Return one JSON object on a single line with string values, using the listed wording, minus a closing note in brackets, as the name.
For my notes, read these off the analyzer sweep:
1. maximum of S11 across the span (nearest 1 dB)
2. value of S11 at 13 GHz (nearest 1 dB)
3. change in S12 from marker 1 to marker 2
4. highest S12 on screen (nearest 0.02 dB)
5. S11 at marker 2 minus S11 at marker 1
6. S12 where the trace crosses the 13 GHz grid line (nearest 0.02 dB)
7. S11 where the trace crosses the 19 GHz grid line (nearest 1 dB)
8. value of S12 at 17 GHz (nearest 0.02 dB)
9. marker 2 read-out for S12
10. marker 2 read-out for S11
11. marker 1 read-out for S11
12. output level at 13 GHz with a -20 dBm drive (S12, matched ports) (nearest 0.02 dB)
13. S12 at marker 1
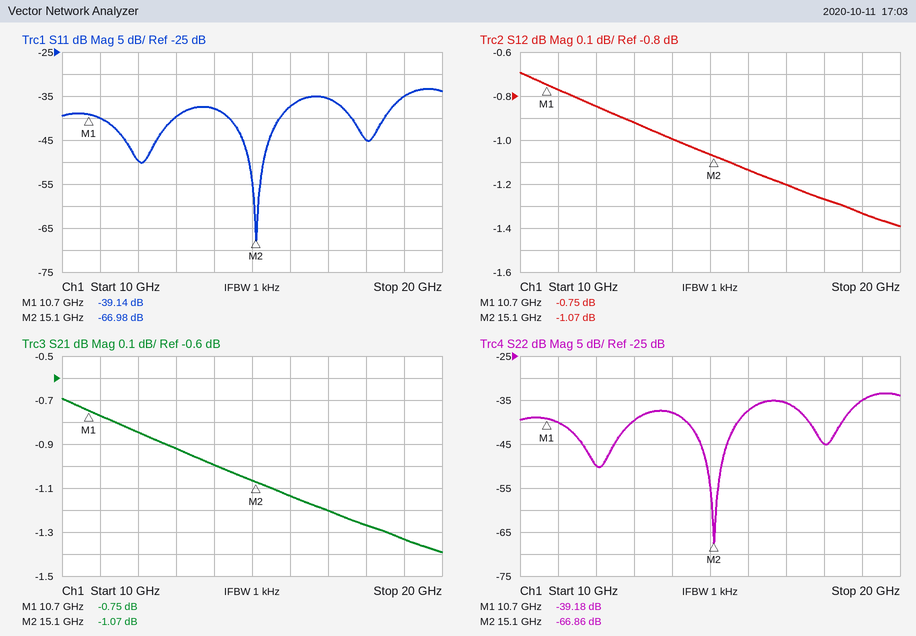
{"maximum of S11 across the span": "-33 dB", "value of S11 at 13 GHz": "-40 dB", "change in S12 from marker 1 to marker 2": "-0.32 dB", "highest S12 on screen": "-0.70 dB", "S11 at marker 2 minus S11 at marker 1": "-27.84 dB", "S12 where the trace crosses the 13 GHz grid line": "-0.92 dB", "S11 where the trace crosses the 19 GHz grid line": "-35 dB", "value of S12 at 17 GHz": "-1.20 dB", "marker 2 read-out for S12": "-1.07 dB", "marker 2 read-out for S11": "-66.98 dB", "marker 1 read-out for S11": "-39.14 dB", "output level at 13 GHz with a -20 dBm drive (S12, matched ports)": "-20.92 dBm", "S12 at marker 1": "-0.75 dB"}
